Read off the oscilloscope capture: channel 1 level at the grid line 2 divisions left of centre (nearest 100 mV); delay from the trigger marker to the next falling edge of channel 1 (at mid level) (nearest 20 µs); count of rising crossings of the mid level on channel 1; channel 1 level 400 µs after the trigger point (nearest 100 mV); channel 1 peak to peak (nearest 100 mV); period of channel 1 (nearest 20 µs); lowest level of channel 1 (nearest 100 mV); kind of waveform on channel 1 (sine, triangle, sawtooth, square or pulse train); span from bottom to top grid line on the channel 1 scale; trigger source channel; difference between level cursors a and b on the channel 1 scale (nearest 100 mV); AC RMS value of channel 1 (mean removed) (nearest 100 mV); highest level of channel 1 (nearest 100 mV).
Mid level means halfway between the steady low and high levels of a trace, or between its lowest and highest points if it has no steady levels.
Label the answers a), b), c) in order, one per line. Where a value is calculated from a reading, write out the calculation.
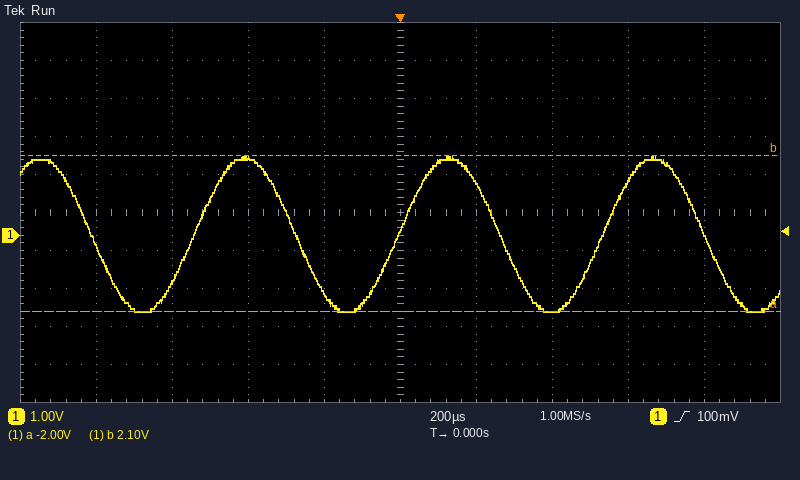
a) 2.0 V
b) 260 µs
c) 3
d) -2.0 V
e) 2.1 V − (-2.0 V) = 4.1 V
f) 540 µs
g) -2.0 V
h) sine
i) 10 V
j) channel 1
k) 4.1 V
l) 4.1 V / (2√2) ≈ 1.4 V
m) 2.1 V
